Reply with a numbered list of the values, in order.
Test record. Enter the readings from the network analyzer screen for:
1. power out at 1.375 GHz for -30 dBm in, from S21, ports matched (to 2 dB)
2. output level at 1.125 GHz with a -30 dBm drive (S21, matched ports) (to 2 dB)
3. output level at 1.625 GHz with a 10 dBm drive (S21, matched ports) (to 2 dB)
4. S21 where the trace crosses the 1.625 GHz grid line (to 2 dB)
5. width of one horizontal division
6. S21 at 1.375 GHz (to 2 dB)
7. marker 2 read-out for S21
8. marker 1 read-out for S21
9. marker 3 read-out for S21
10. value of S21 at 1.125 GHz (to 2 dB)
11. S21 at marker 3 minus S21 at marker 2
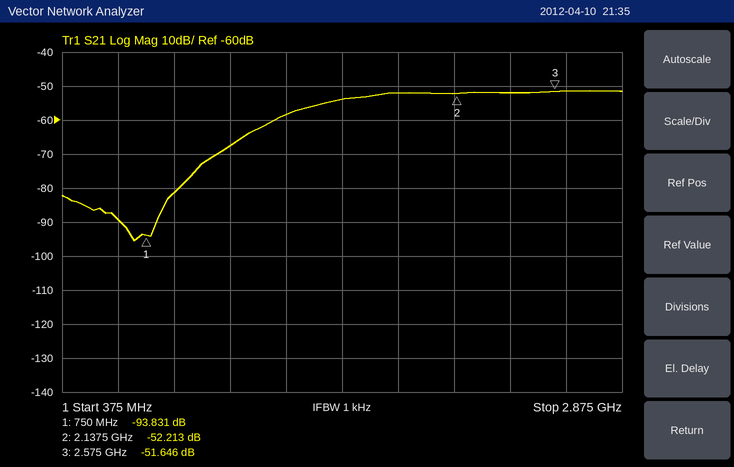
1. -88 dBm
2. -98 dBm
3. -44 dBm
4. -54 dB
5. 250 MHz
6. -58 dB
7. -52.213 dB
8. -93.831 dB
9. -51.646 dB
10. -68 dB
11. 0.567 dB
